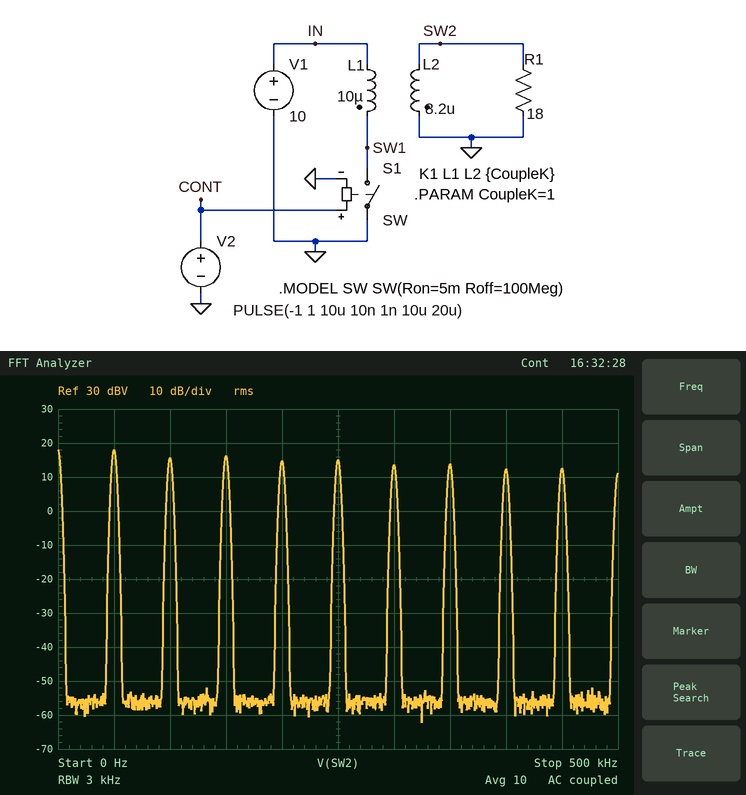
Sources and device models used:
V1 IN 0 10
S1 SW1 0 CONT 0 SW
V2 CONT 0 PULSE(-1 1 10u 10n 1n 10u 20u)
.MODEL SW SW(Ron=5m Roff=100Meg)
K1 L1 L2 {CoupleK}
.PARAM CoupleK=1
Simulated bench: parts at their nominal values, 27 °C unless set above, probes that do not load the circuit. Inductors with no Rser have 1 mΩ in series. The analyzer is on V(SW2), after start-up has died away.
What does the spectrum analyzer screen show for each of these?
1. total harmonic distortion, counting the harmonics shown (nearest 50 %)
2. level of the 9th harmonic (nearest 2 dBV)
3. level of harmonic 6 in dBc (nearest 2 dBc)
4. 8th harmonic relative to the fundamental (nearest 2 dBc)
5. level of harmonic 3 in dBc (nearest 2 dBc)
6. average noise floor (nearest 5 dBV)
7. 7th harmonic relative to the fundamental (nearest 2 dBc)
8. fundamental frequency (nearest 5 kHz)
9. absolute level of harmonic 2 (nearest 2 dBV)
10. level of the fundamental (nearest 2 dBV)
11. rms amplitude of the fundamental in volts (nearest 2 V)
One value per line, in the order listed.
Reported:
200 %
12 dBV
-4 dBc
-6 dBc
-2 dBc
-55 dBV
-4 dBc
50 kHz
16 dBV
18 dBV
8 V
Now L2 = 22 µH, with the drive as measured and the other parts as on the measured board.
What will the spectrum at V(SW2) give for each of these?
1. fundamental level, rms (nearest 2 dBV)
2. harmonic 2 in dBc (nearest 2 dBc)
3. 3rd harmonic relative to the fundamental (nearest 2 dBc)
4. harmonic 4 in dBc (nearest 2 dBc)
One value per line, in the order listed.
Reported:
22 dBV
-4 dBc
-4 dBc
-8 dBc
